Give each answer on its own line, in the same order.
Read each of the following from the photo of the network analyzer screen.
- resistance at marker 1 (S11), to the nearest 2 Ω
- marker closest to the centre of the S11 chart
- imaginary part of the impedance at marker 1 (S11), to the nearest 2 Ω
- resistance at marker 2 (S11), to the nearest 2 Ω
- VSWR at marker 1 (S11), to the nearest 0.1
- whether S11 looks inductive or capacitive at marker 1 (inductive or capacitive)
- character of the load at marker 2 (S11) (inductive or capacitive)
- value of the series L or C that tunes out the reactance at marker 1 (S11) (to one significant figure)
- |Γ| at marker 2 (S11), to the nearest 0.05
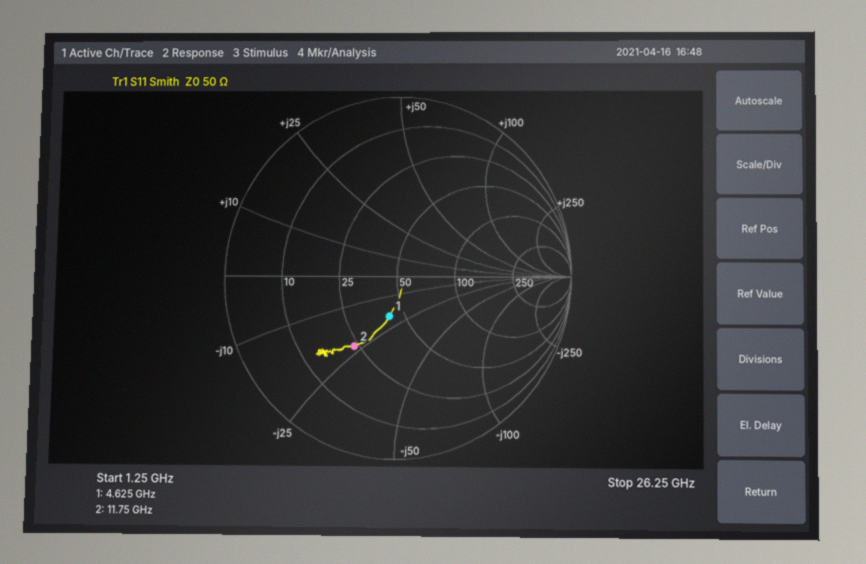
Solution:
42 Ω
marker 1
-20 Ω
24 Ω
1.6
capacitive
capacitive
700 pH
0.45
